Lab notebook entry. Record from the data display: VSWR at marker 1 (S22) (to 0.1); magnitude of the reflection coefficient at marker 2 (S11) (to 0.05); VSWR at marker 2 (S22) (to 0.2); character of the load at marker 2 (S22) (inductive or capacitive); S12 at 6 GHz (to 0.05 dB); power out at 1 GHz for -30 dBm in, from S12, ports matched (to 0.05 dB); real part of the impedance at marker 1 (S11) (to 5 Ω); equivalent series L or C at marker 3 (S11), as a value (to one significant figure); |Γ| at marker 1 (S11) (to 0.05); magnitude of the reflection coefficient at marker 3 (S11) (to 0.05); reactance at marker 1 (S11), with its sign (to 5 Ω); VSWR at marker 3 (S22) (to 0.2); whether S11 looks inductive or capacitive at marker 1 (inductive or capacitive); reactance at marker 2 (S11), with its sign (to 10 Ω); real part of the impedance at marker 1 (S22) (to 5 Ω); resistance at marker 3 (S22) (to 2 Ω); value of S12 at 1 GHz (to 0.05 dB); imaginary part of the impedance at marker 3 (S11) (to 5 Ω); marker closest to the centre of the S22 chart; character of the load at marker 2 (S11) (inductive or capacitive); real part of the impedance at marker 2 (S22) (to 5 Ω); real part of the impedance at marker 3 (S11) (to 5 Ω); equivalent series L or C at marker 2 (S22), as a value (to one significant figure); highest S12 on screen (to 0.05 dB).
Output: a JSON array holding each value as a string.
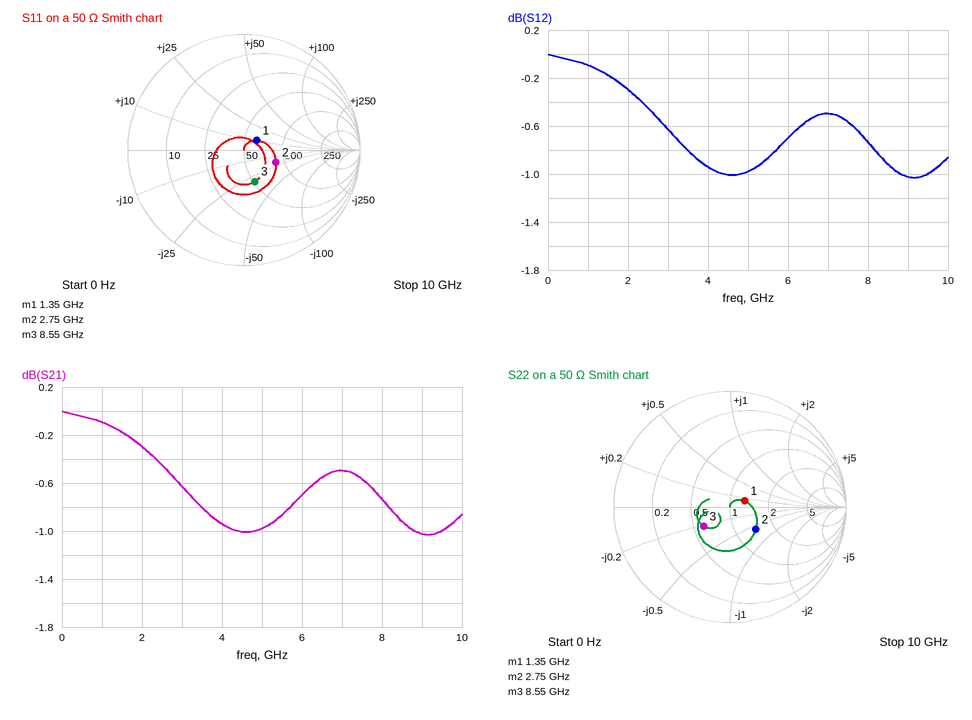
["1.3", "0.30", "1.8", "capacitive", "-0.70 dB", "-30.10 dBm", "60 Ω", "600 fF", "0.15", "0.30", "+10 Ω", "1.8", "inductive", "-20 Ω", "65 Ω", "30 Ω", "-0.10 dB", "-30 Ω", "marker 1", "capacitive", "70 Ω", "50 Ω", "2 pF", "0.00 dB"]
